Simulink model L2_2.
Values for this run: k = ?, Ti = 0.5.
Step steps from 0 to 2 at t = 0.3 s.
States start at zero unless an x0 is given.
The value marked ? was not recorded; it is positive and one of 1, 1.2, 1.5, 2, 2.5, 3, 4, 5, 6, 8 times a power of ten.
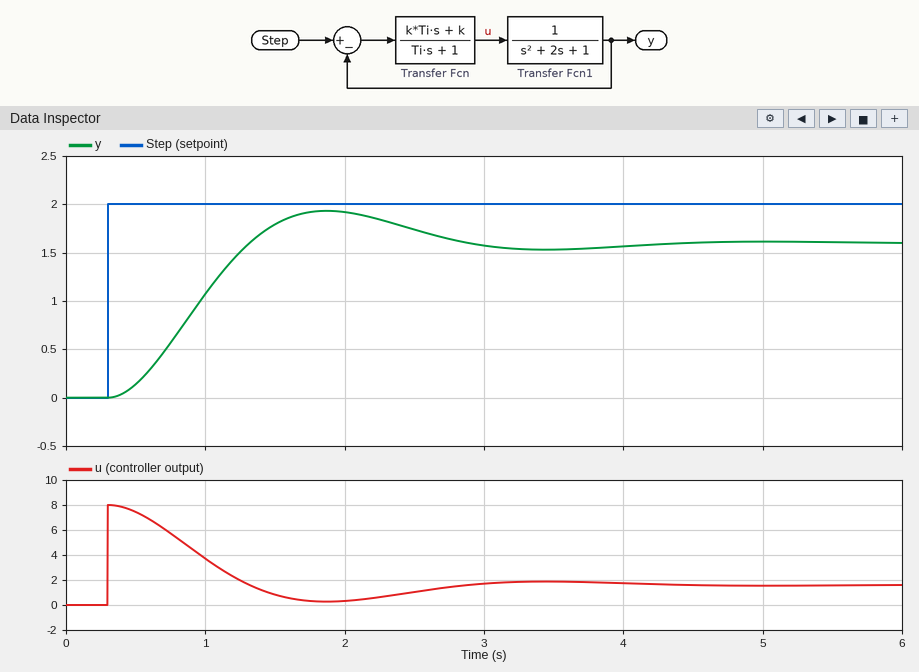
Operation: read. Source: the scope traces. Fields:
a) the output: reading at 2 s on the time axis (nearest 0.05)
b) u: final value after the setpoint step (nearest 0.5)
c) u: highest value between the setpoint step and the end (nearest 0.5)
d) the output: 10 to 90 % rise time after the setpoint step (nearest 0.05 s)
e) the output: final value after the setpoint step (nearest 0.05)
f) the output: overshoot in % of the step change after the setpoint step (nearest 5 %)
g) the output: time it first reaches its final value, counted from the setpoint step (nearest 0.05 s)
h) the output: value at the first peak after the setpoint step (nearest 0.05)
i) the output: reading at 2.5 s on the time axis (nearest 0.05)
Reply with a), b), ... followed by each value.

a) 1.90
b) 1.5
c) 8.0
d) 0.70 s
e) 1.60
f) 20 %
g) 1.00 s
h) 1.95
i) 1.75
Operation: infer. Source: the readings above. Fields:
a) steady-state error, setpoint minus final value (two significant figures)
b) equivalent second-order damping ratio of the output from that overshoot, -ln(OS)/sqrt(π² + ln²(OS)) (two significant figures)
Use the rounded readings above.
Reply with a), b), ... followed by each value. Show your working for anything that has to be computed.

a) 2 - 1.6 = 0.40
b) ln(0.2) = -1.609; 1.609 / sqrt(9.870 + 2.590) = 0.46
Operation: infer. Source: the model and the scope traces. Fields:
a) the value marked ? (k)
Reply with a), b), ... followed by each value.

a) 4
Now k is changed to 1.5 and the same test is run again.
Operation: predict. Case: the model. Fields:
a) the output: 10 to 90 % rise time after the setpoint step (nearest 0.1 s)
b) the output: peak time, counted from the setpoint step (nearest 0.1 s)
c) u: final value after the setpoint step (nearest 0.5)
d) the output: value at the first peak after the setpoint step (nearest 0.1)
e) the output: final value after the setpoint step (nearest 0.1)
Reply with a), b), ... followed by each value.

a) 1.2 s
b) 2.6 s
c) 1.0
d) 1.3
e) 1.2
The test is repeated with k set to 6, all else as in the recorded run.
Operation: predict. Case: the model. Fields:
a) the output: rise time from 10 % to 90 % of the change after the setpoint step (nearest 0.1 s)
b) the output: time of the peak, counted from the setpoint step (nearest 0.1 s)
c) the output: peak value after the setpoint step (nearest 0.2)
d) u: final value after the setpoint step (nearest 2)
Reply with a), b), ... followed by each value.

a) 0.5 s
b) 1.3 s
c) 2.2
d) 2
